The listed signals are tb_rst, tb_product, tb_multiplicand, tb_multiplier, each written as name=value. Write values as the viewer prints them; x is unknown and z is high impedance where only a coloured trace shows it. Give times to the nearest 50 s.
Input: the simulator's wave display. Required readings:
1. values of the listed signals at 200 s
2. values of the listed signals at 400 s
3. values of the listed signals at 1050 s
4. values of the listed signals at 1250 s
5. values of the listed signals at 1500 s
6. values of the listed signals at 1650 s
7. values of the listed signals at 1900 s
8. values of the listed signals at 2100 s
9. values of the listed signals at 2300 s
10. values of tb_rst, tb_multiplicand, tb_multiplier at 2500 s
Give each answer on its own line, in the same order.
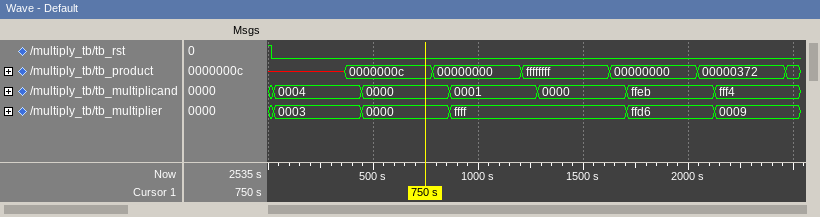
tb_rst=0, tb_product=x, tb_multiplicand=0004, tb_multiplier=0003
tb_rst=0, tb_product=0000000c, tb_multiplicand=0004, tb_multiplier=0003
tb_rst=0, tb_product=00000000, tb_multiplicand=0001, tb_multiplier=ffff
tb_rst=0, tb_product=ffffffff, tb_multiplicand=0001, tb_multiplier=ffff
tb_rst=0, tb_product=ffffffff, tb_multiplicand=0000, tb_multiplier=ffff
tb_rst=0, tb_product=00000000, tb_multiplicand=0000, tb_multiplier=ffff
tb_rst=0, tb_product=00000000, tb_multiplicand=ffeb, tb_multiplier=ffd6
tb_rst=0, tb_product=00000372, tb_multiplicand=ffeb, tb_multiplier=ffd6
tb_rst=0, tb_product=00000372, tb_multiplicand=fff4, tb_multiplier=0009
tb_rst=0, tb_multiplicand=fff4, tb_multiplier=0009
